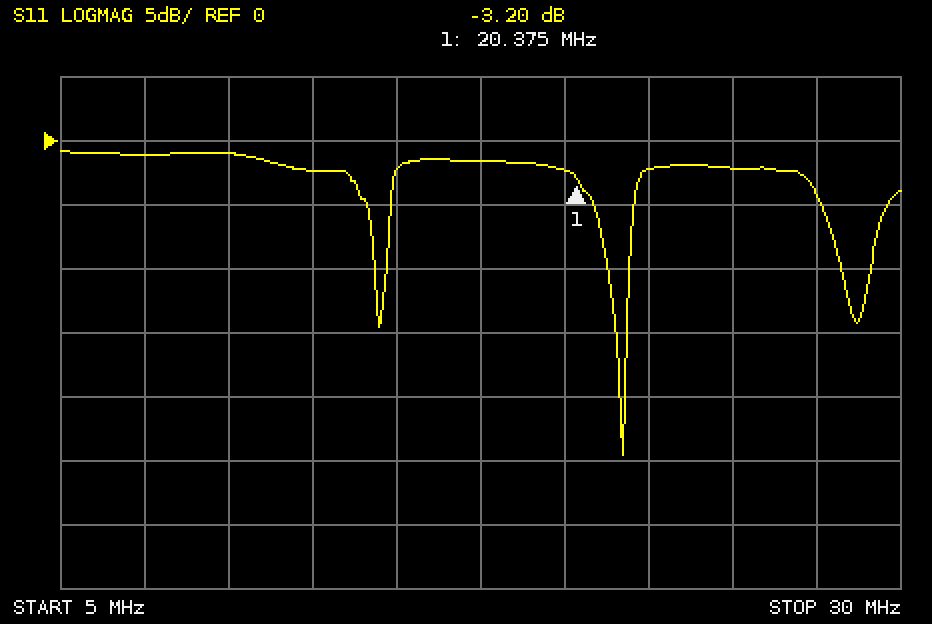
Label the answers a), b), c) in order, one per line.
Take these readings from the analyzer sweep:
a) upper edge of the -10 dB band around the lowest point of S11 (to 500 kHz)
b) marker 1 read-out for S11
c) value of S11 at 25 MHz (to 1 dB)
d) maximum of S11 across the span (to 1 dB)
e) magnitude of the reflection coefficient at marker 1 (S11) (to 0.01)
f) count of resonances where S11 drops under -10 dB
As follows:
a) 22.0 MHz
b) -3.20 dB
c) -2 dB
d) -1 dB
e) 0.69
f) 3
